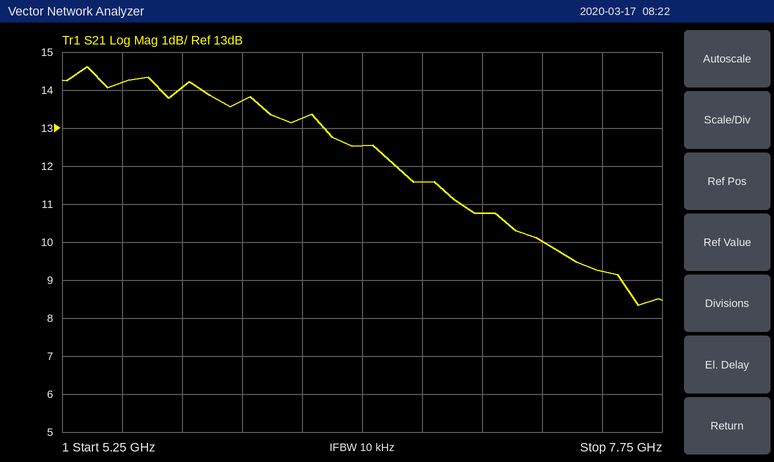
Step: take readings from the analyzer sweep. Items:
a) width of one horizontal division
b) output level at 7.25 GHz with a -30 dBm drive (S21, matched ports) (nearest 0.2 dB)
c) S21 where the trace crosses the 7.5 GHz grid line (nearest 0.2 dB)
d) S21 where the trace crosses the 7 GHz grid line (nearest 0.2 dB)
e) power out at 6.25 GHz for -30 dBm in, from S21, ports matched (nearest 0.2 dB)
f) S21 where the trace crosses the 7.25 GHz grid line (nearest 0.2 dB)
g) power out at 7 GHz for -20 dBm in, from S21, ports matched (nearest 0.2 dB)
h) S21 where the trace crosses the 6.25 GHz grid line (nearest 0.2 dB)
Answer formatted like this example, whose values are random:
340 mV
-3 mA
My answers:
250 MHz
-20.0 dBm
9.2 dB
10.8 dB
-16.8 dBm
10.0 dB
-9.2 dBm
13.2 dB
